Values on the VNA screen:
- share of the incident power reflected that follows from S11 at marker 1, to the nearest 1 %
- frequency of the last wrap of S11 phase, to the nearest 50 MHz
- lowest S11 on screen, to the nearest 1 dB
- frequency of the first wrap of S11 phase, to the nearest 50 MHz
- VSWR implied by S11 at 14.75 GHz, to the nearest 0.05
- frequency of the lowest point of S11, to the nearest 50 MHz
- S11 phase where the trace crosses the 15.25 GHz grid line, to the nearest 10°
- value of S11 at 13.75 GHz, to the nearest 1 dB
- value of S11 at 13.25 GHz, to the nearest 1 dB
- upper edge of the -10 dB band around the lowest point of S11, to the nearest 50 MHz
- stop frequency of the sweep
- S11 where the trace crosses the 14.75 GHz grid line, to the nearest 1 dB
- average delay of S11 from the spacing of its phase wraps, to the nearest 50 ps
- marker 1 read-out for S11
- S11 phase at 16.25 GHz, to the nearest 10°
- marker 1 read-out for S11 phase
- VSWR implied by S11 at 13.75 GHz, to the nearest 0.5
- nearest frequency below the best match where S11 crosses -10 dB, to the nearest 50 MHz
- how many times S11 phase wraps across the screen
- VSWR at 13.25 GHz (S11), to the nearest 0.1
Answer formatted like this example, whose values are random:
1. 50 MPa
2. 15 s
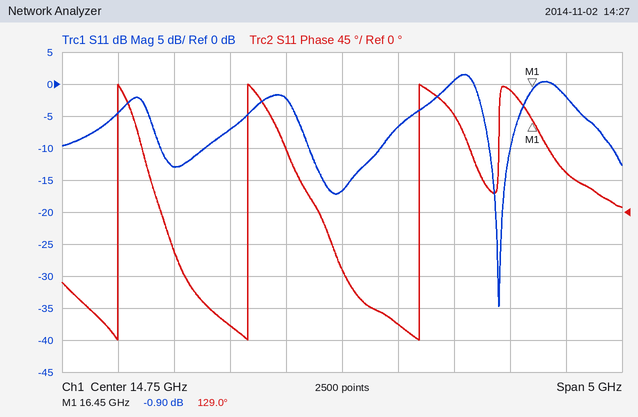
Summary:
1. 81 %
2. 15.45 GHz
3. -35 dB
4. 12.75 GHz
5. 1.35
6. 16.15 GHz
7. -160°
8. -7 dB
9. -13 dB
10. 16.25 GHz
11. 17.25 GHz
12. -17 dB
13. 750 ps
14. -0.90 dB
15. 170°
16. 129.0°
17. 2.5
18. 16.05 GHz
19. 3
20. 1.6
